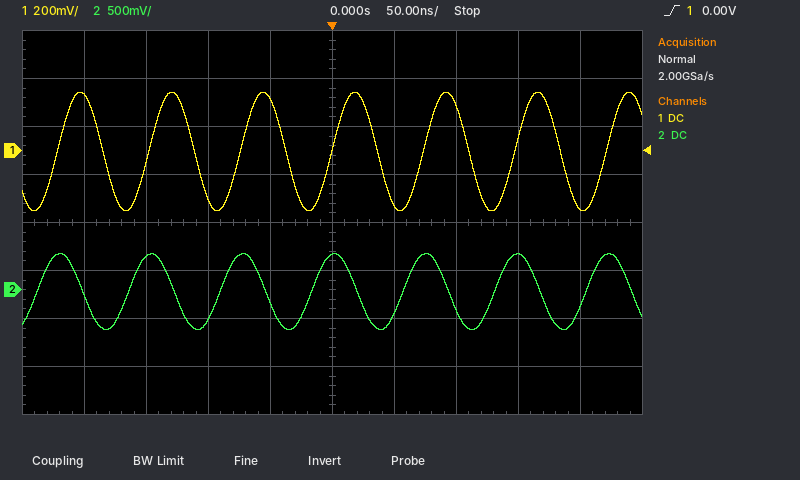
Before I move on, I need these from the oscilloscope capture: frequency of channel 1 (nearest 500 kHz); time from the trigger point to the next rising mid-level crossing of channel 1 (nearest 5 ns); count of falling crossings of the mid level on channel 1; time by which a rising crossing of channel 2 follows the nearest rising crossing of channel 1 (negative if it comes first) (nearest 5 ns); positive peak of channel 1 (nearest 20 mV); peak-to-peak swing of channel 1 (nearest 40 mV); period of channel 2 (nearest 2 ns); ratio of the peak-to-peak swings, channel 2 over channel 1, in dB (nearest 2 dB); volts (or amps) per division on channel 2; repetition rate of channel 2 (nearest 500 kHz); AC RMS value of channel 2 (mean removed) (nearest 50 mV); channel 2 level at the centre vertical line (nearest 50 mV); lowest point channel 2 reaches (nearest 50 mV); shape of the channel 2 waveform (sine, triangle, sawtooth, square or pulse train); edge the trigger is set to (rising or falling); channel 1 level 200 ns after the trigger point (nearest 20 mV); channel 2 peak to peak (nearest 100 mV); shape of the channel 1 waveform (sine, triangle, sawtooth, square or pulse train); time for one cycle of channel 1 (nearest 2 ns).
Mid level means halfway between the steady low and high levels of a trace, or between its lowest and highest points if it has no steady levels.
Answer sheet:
13.5 MHz
75 ns
6
-15 ns
240 mV
480 mV
74 ns
4 dB
500 mV
13.5 MHz
300 mV
350 mV
-400 mV
sine
rising
-240 mV
800 mV
sine
74 ns
